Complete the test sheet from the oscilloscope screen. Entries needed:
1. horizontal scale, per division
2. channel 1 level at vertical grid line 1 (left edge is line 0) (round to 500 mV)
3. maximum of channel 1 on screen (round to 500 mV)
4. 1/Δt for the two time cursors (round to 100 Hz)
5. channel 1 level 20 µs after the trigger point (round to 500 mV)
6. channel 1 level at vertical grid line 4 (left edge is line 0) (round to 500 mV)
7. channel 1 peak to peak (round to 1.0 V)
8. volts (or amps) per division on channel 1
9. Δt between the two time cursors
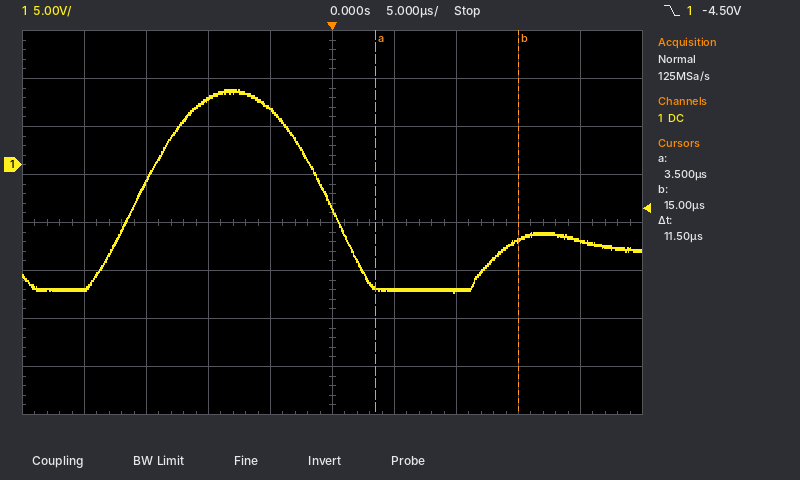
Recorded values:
5 µs
-13.0 V
8.0 V
87.0 kHz
-8.0 V
6.0 V
21.0 V
5 V
11.5 µs
